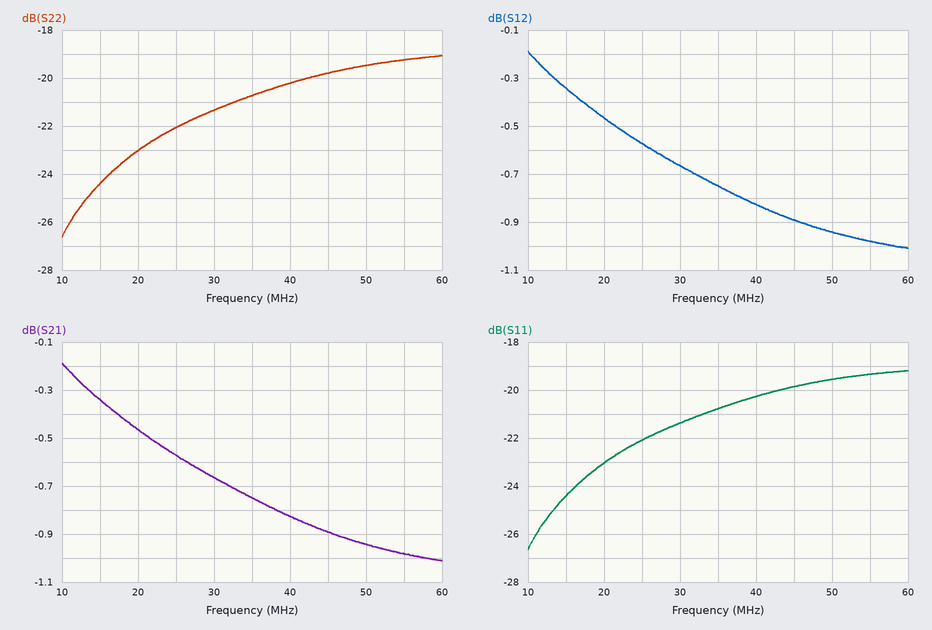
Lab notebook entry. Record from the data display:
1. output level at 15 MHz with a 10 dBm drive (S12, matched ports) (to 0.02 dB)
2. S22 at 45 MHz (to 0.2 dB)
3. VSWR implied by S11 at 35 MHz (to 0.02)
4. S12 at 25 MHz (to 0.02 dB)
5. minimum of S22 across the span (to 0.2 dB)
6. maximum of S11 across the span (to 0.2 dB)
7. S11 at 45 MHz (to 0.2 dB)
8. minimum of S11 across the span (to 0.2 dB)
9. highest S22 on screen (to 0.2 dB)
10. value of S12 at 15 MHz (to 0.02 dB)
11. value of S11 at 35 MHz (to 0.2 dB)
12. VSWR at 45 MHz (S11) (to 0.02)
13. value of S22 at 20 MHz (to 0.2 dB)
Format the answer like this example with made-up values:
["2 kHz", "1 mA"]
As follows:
["9.66 dBm", "-19.8 dB", "1.20", "-0.58 dB", "-26.6 dB", "-19.2 dB", "-19.8 dB", "-26.6 dB", "-19.0 dB", "-0.34 dB", "-20.8 dB", "1.22", "-23.0 dB"]
